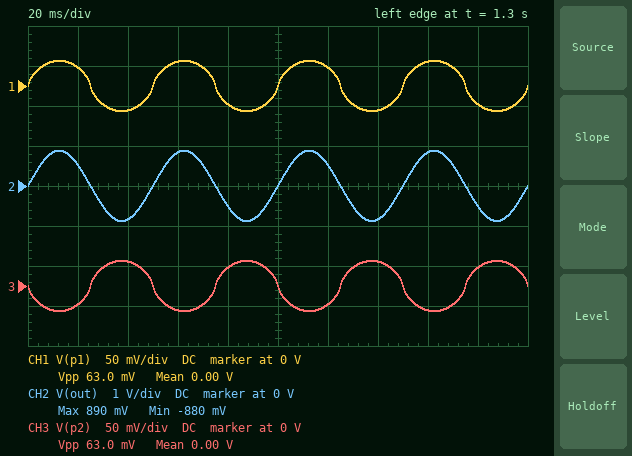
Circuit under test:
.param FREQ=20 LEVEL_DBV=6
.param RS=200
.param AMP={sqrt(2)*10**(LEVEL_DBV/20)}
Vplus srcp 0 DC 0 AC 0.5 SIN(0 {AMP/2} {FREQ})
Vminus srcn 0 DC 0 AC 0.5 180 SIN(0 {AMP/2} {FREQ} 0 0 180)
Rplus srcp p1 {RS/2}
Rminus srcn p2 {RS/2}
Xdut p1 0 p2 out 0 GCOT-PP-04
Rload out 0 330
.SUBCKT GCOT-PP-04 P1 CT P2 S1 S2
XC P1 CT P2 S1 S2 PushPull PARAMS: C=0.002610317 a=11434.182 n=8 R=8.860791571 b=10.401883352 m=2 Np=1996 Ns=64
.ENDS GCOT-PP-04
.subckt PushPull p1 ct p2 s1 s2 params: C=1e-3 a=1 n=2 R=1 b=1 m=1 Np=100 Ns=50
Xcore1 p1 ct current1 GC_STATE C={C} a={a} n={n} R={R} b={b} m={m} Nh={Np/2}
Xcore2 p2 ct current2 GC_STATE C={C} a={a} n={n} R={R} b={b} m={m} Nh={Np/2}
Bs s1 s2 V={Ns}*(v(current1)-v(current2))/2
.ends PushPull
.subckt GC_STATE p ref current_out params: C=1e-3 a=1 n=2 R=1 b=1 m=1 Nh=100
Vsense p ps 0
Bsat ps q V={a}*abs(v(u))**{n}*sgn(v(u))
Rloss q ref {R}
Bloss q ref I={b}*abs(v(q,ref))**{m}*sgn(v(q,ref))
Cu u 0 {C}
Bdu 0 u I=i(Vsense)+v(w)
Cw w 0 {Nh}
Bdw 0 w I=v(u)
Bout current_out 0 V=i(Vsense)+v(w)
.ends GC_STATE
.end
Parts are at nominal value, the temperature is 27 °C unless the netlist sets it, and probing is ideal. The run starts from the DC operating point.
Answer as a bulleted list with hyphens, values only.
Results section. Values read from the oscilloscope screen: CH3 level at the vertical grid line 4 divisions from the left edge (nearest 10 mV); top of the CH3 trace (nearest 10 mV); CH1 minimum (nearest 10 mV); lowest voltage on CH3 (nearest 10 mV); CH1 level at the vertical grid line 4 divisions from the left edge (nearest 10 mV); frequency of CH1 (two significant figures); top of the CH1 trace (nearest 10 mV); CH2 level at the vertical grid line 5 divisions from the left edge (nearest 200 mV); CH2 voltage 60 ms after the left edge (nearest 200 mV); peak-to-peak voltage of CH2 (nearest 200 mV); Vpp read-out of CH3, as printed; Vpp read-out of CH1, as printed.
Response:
- 20 mV
- 30 mV
- -30 mV
- -30 mV
- -20 mV
- 20 Hz
- 30 mV
- 0 V
- 800 mV
- 1.8 V
- 63.0 mV
- 63.0 mV
